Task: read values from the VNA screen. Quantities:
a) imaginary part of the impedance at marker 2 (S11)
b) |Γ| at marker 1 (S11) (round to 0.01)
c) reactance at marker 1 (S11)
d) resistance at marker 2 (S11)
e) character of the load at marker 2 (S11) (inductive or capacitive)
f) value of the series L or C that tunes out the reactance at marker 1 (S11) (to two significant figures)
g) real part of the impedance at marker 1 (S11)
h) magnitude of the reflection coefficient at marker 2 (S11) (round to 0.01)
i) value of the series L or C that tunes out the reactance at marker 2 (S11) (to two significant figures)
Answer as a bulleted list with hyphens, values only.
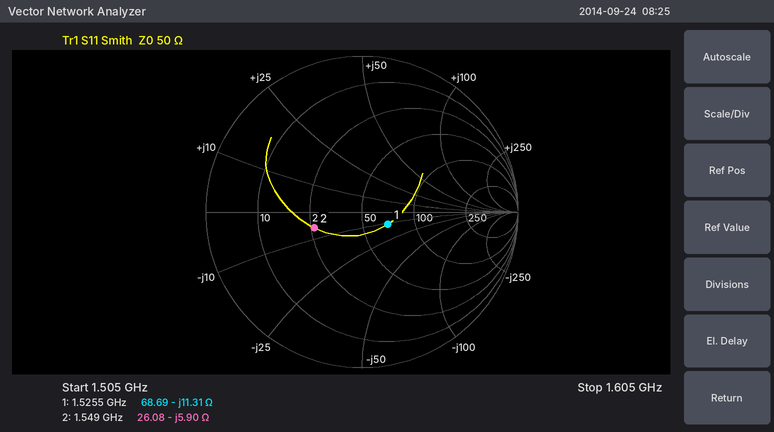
- -5.90 Ω
- 0.18
- -11.31 Ω
- 26.08 Ω
- capacitive
- 1.2 nH
- 68.69 Ω
- 0.32
- 610 pH
